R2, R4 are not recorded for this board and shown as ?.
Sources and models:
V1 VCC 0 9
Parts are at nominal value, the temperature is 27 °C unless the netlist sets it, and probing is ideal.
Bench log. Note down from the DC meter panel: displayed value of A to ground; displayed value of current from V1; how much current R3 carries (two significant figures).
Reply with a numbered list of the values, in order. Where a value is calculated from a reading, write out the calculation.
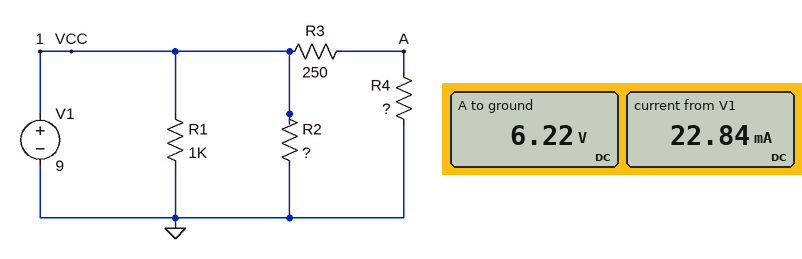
1. 6.22 V
2. 22.84 mA
3. (9 V - 6.22 V) / 250 Ω = 11 mA
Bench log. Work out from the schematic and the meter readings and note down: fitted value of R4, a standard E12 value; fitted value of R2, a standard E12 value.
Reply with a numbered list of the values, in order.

1. 560 Ω
2. 3.3 kΩ
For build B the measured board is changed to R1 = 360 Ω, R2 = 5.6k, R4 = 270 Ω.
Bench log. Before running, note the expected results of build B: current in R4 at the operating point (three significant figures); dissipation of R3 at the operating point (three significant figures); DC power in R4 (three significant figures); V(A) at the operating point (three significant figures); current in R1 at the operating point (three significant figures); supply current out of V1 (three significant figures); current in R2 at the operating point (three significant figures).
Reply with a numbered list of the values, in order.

1. 17.3 mA
2. 74.9 mW
3. 80.9 mW
4. 4.67 V
5. 25.0 mA
6. 43.9 mA
7. 1.61 mA
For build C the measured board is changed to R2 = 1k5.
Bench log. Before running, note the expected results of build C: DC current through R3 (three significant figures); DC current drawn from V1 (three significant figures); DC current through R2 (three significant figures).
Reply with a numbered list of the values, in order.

1. 11.1 mA
2. 26.1 mA
3. 6.00 mA
